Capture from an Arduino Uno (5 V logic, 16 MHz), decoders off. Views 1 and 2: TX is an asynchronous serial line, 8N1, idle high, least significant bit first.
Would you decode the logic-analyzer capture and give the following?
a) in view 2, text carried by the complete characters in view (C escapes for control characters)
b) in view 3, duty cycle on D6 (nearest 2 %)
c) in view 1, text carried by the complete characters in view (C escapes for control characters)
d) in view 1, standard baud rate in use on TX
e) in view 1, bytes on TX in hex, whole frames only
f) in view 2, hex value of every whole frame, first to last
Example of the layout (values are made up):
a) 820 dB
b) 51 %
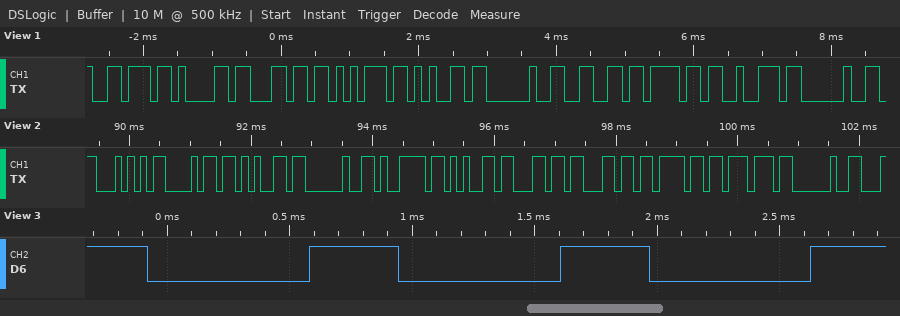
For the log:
a) "The yellow "
b) 36 %
c) "value for "
d) 9600 baud
e) 76 61 6C 75 65 20 66 6F 72 20
f) 54 68 65 20 79 65 6C 6C 6F 77 20
